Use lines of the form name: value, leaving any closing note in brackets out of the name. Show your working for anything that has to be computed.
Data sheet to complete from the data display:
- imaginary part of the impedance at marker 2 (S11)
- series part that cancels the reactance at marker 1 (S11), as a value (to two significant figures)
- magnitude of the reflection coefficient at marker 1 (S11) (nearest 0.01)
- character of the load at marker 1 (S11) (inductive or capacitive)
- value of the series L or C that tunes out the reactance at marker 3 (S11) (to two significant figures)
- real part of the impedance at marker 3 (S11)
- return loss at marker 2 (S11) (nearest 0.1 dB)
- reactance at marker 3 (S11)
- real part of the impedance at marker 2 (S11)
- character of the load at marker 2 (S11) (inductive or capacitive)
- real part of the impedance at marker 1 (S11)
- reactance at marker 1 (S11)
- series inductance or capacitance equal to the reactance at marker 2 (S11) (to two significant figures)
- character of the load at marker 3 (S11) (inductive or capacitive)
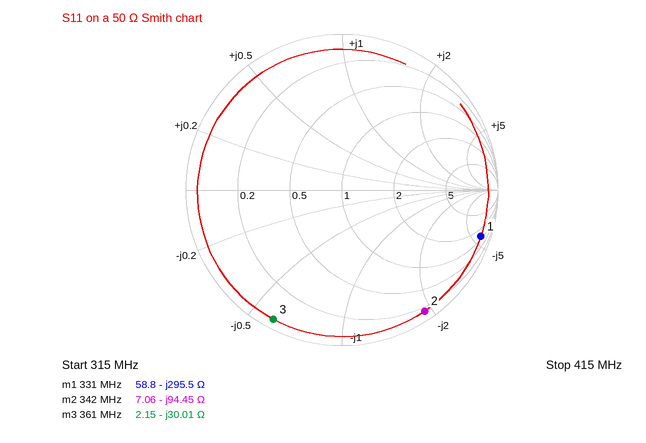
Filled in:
imaginary part of the impedance at marker 2: -94.45 Ω
series part that cancels the reactance at marker 1 (S11), as a value: L = 295.5 Ω/(2π × 331 MHz) ≈ 142 nH, so 140 nH to two significant figures
magnitude of the reflection coefficient at marker 1 (S11): 0.94
character of the load at marker 1 (S11): capacitive
value of the series L or C that tunes out the reactance at marker 3 (S11): L = 30.01 Ω/(2π × 361 MHz) ≈ 13 nH
real part of the impedance at marker 3: 2.15 Ω
return loss at marker 2 (S11): 0.5 dB
reactance at marker 3: -30.01 Ω
real part of the impedance at marker 2: 7.06 Ω
character of the load at marker 2 (S11): capacitive
real part of the impedance at marker 1: 58.8 Ω
reactance at marker 1: -295.5 Ω
series inductance or capacitance equal to the reactance at marker 2 (S11): C = 1/(2π × 342 MHz × 94.45 Ω) ≈ 4.9 pF
character of the load at marker 3 (S11): capacitive
